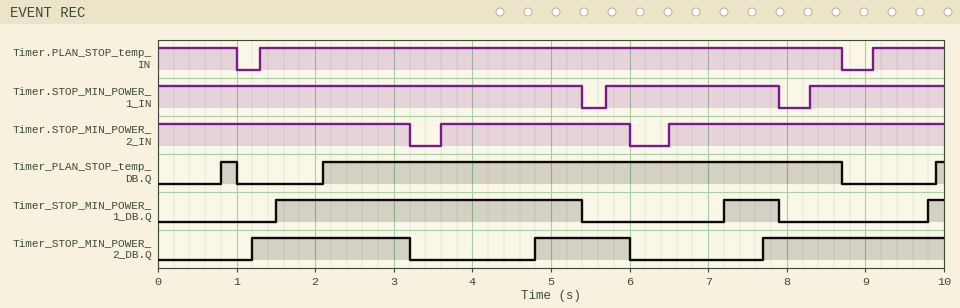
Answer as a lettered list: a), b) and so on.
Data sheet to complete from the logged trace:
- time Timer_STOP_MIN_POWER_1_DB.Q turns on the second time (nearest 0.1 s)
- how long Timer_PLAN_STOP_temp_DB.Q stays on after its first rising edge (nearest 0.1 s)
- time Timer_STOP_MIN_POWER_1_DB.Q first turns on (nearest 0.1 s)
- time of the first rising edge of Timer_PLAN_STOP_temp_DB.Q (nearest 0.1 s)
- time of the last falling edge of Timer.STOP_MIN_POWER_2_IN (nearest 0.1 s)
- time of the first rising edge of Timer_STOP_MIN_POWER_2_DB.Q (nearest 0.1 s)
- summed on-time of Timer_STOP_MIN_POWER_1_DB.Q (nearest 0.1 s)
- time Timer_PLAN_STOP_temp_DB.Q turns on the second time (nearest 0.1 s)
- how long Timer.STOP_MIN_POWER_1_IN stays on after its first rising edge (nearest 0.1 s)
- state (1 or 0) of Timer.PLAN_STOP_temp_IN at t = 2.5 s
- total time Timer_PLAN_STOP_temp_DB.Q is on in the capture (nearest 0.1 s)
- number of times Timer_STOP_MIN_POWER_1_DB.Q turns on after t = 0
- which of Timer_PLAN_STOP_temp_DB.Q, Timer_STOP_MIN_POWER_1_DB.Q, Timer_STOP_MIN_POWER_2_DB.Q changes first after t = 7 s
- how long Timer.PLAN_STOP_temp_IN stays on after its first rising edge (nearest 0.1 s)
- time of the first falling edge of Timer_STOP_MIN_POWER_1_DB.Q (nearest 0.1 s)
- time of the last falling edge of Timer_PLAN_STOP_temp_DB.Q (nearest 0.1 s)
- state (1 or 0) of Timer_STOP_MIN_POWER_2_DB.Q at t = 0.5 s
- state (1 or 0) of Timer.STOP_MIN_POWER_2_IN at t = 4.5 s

a) 7.2 s
b) 0.2 s
c) 1.5 s
d) 0.8 s
e) 6.0 s
f) 1.2 s
g) 4.8 s
h) 2.1 s
i) 2.2 s
j) 1
k) 6.9 s
l) 3
m) Timer_STOP_MIN_POWER_1_DB.Q
n) 7.4 s
o) 5.4 s
p) 8.7 s
q) 0
r) 1
